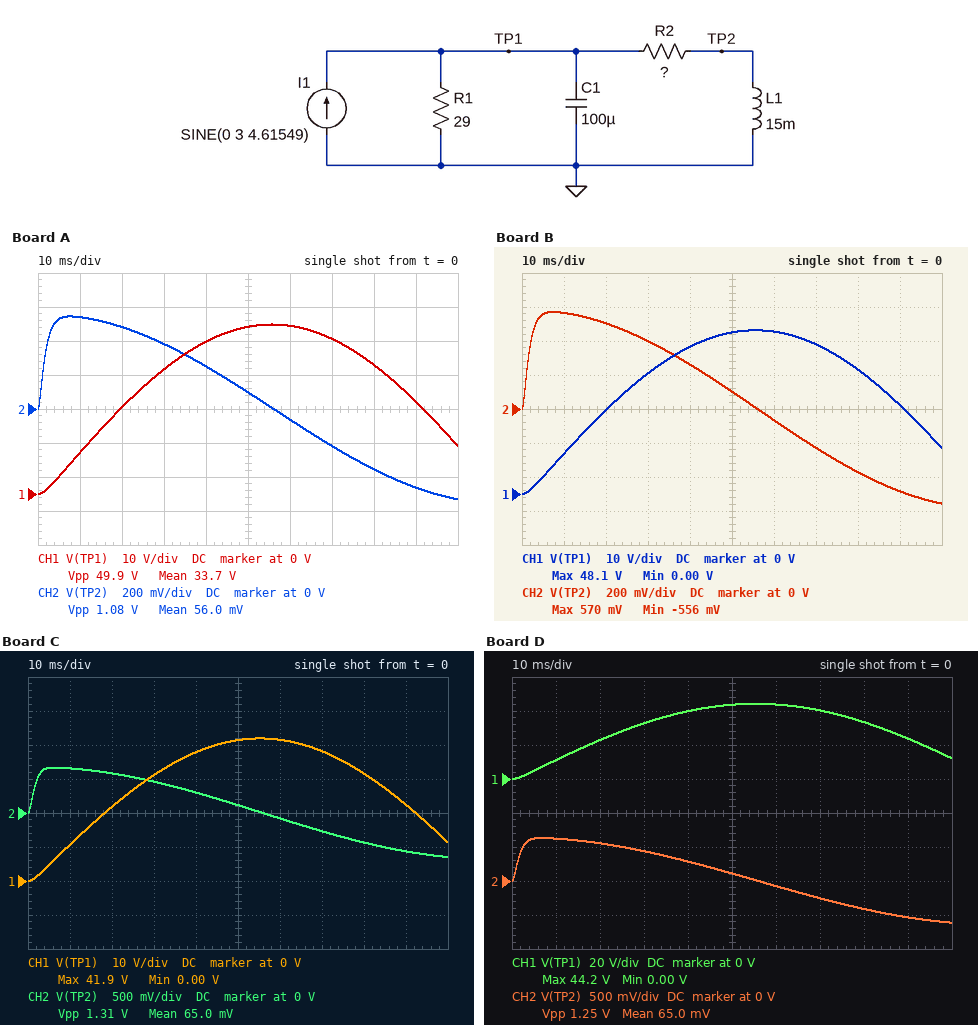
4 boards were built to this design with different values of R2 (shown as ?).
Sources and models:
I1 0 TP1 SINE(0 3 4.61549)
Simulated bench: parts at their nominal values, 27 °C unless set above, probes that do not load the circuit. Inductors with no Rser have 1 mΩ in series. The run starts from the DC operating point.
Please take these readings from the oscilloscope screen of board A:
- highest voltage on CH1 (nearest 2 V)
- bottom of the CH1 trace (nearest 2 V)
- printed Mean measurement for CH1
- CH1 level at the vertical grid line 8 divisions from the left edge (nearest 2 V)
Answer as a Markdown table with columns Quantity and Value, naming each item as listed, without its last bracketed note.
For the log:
| Quantity | Value |
|---|---|
| highest voltage on CH1 | 50 V |
| bottom of the CH1 trace | 0 V |
| printed Mean measurement for CH1 | 33.7 V |
| CH1 level at the vertical grid line 8 divisions from the left edge | 38 V |
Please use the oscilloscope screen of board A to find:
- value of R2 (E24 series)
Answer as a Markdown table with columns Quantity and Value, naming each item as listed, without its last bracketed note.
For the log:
| Quantity | Value |
|---|---|
| value of R2 | 39 Ω |
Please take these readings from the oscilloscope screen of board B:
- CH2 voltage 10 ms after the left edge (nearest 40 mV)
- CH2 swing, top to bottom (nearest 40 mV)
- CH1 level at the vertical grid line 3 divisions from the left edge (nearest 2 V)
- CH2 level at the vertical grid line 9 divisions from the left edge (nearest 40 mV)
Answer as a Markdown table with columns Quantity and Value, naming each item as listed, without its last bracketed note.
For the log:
| Quantity | Value |
|---|---|
| CH2 voltage 10 ms after the left edge | 560 mV |
| CH2 swing, top to bottom | 1.12 V |
| CH1 level at the vertical grid line 3 divisions from the left edge | 36 V |
| CH2 level at the vertical grid line 9 divisions from the left edge | -480 mV |
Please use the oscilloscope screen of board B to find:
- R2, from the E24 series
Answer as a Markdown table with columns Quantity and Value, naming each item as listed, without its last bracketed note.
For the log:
| Quantity | Value |
|---|---|
| R2, from the E24 series | 36 Ω |
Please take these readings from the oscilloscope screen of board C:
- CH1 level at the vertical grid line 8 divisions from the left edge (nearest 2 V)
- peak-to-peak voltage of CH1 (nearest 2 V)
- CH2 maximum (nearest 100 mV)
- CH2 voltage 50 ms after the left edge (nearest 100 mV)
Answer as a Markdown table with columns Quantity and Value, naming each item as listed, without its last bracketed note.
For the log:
| Quantity | Value |
|---|---|
| CH1 level at the vertical grid line 8 divisions from the left edge | 32 V |
| peak-to-peak voltage of CH1 | 42 V |
| CH2 maximum | 700 mV |
| CH2 voltage 50 ms after the left edge | 100 mV |
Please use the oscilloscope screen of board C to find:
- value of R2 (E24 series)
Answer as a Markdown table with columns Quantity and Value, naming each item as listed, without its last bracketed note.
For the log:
| Quantity | Value |
|---|---|
| value of R2 | 27 Ω |
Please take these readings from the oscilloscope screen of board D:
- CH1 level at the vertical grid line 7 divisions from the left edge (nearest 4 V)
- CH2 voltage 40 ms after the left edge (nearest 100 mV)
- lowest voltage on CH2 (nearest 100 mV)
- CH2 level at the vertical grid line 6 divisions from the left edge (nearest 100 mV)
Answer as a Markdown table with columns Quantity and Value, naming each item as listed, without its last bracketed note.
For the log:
| Quantity | Value |
|---|---|
| CH1 level at the vertical grid line 7 divisions from the left edge | 40 V |
| CH2 voltage 40 ms after the left edge | 300 mV |
| lowest voltage on CH2 | -600 mV |
| CH2 level at the vertical grid line 6 divisions from the left edge | -100 mV |
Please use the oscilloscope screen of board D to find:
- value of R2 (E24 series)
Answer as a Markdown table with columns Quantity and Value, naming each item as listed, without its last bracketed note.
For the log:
| Quantity | Value |
|---|---|
| value of R2 | 30 Ω |
